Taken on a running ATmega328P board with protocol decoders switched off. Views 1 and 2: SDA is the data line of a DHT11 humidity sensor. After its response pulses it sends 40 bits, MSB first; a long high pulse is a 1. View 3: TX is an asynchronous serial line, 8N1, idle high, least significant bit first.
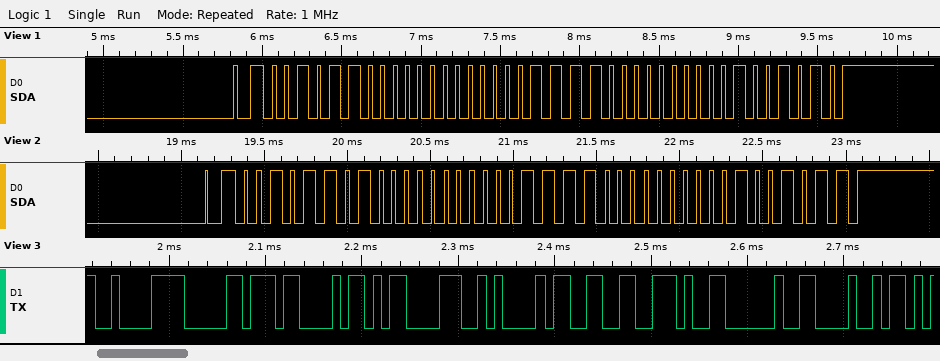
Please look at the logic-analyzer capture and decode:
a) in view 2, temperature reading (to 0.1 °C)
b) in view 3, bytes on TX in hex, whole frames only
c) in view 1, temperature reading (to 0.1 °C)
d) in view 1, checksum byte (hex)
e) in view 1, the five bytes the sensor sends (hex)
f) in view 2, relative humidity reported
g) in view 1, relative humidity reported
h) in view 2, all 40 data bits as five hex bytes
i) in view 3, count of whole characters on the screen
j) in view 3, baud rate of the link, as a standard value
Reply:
30.0 °C
C2 B0 43 0D 0A 33 2E 20 48
30.0 °C
0x4A
2C 00 1E 00 4A
45 %
44 %
2D 00 1E 00 4B
9
115200 baud
